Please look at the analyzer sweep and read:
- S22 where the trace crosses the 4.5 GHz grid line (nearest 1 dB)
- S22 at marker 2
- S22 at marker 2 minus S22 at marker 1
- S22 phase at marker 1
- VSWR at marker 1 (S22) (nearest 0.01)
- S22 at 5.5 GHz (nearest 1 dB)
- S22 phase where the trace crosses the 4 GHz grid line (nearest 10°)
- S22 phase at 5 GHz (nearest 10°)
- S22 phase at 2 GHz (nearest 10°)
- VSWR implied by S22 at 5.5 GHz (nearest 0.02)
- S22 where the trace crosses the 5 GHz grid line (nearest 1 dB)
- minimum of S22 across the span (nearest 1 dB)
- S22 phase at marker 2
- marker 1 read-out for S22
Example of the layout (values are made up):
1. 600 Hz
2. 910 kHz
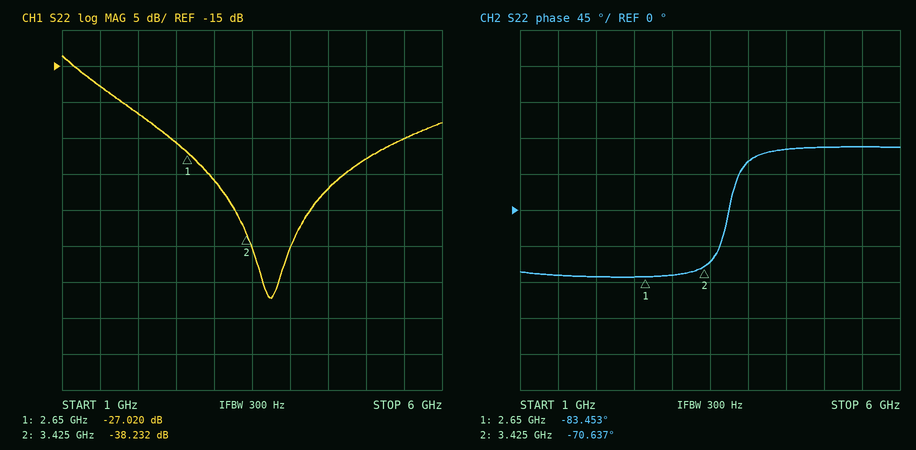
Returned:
1. -32 dB
2. -38.232 dB
3. -11.212 dB
4. -83.453°
5. 1.09
6. -25 dB
7. 60°
8. 80°
9. -80°
10. 1.12
11. -28 dB
12. -47 dB
13. -70.637°
14. -27.020 dB
